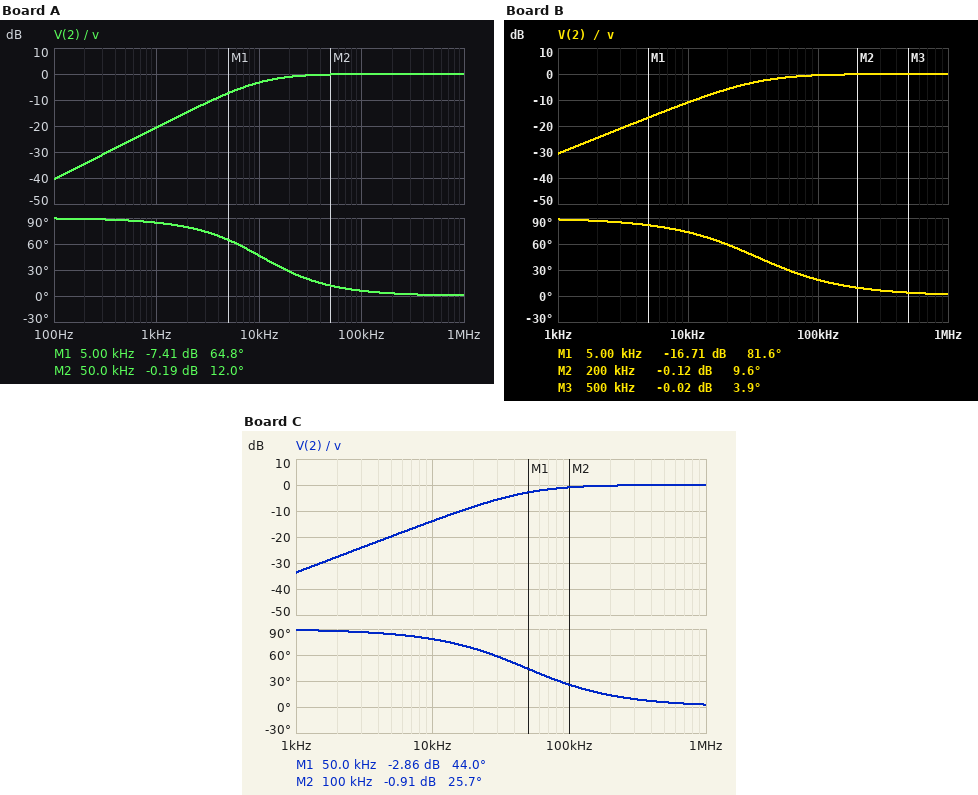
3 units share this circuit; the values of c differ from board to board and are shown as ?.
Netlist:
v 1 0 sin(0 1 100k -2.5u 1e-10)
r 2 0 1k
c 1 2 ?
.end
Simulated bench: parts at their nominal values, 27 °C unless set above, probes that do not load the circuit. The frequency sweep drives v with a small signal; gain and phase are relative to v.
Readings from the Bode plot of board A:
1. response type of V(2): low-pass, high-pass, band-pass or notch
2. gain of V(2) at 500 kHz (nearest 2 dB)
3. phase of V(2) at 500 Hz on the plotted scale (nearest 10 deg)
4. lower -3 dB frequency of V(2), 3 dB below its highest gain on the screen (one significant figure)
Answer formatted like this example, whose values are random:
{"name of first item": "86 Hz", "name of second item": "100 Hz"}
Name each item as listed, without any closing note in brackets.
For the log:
{"response type of V(2): low-pass, high-pass, band-pass or notch": "high-pass", "gain of V(2) at 500 kHz": "0 dB", "phase of V(2) at 500 Hz on the plotted scale": "90 deg", "lower -3 dB frequency of V(2), 3 dB below its highest gain on the screen": "10 kHz"}
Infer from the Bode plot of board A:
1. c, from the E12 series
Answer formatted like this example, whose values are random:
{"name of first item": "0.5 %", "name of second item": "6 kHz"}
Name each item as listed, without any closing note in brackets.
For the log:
{"c, from the E12 series": "15 nF"}
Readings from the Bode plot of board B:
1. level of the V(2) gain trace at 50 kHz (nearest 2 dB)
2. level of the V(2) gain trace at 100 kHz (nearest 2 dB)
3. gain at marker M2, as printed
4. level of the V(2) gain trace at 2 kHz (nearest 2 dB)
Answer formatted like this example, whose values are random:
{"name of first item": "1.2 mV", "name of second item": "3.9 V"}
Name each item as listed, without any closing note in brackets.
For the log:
{"level of the V(2) gain trace at 50 kHz": "-2 dB", "level of the V(2) gain trace at 100 kHz": "0 dB", "gain at marker M2, as printed": "-0.12 dB", "level of the V(2) gain trace at 2 kHz": "-24 dB"}
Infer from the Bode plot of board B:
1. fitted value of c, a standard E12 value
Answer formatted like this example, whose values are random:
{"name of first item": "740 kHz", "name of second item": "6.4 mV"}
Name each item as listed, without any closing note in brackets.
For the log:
{"fitted value of c, a standard E12 value": "4.7 nF"}
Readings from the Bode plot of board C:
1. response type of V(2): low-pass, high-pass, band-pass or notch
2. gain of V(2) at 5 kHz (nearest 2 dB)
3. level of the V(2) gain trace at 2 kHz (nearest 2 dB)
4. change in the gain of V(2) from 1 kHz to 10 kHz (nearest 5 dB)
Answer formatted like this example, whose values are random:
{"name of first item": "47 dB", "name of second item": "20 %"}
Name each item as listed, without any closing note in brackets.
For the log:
{"response type of V(2): low-pass, high-pass, band-pass or notch": "high-pass", "gain of V(2) at 5 kHz": "-20 dB", "level of the V(2) gain trace at 2 kHz": "-28 dB", "change in the gain of V(2) from 1 kHz to 10 kHz": "20 dB"}
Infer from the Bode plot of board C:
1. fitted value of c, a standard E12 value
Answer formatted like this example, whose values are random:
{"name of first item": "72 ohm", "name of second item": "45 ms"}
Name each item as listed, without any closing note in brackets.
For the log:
{"fitted value of c, a standard E12 value": "3.3 nF"}
